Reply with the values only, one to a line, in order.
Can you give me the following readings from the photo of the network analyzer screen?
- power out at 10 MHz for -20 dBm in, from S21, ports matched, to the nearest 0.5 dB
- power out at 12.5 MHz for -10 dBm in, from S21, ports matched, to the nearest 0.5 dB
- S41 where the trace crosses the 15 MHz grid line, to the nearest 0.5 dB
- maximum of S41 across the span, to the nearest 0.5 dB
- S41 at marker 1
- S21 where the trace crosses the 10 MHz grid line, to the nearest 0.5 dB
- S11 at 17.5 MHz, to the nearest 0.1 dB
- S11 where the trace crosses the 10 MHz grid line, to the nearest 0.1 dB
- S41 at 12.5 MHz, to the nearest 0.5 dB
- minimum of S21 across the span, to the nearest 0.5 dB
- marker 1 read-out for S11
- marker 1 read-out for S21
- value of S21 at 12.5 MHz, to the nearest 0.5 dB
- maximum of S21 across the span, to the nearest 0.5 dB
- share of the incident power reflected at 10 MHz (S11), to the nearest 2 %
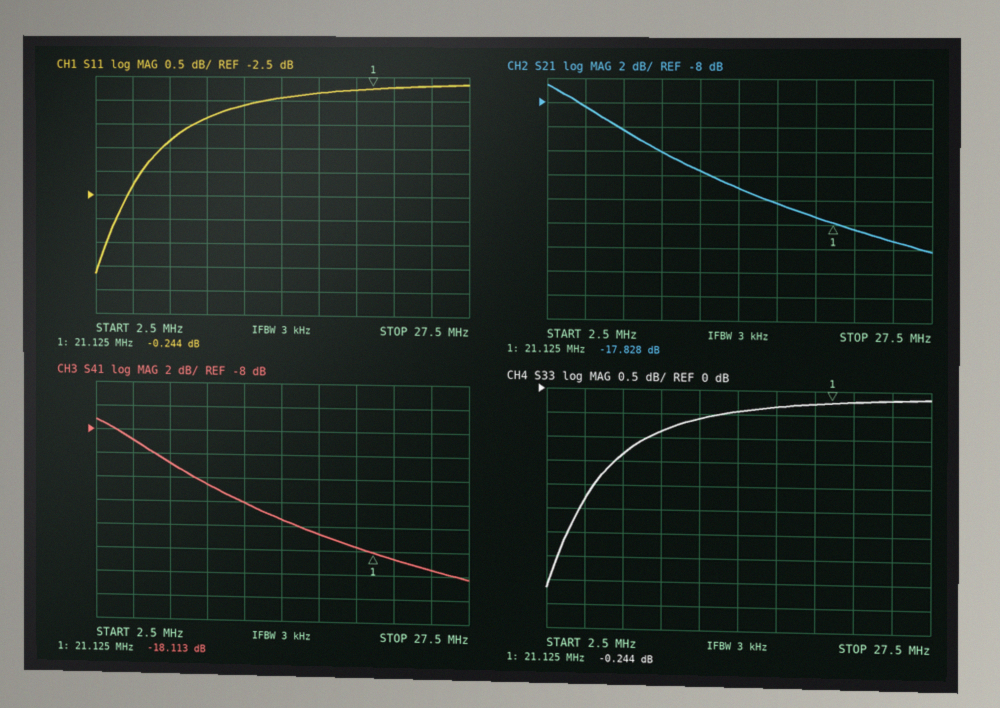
-32.0 dBm
-23.5 dBm
-15.5 dB
-7.0 dB
-18.113 dB
-12.0 dB
-0.3 dB
-0.9 dB
-14.0 dB
-20.0 dB
-0.244 dB
-17.828 dB
-13.5 dB
-6.5 dB
82 %
